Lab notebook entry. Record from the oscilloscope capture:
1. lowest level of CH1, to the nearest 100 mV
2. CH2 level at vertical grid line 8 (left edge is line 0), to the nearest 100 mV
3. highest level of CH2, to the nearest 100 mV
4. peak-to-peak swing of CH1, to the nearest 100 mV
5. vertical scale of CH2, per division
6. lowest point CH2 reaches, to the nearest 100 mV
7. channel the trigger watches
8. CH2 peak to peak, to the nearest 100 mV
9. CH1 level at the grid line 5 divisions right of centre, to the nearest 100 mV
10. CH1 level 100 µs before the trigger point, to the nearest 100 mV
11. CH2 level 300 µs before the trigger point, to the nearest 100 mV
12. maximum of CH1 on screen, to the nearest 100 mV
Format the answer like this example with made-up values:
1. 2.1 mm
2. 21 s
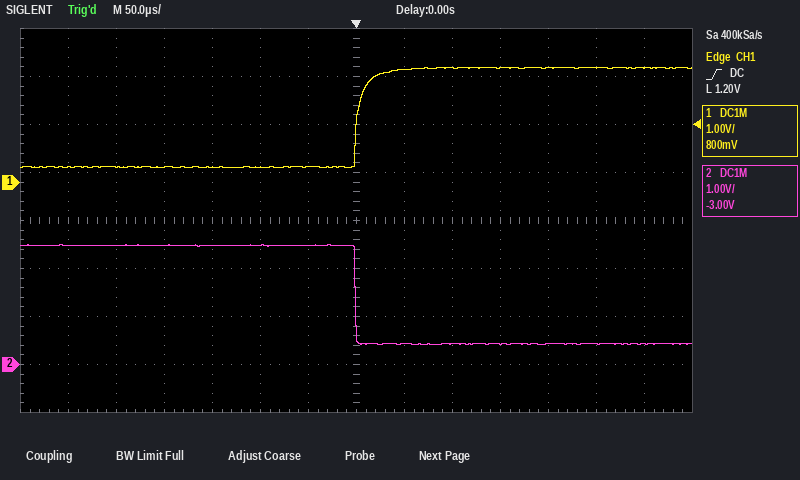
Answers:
1. 300 mV
2. 400 mV
3. 2.5 V
4. 2.1 V
5. 1 V
6. 400 mV
7. CH1
8. 2.1 V
9. 2.4 V
10. 300 mV
11. 2.5 V
12. 2.4 V
